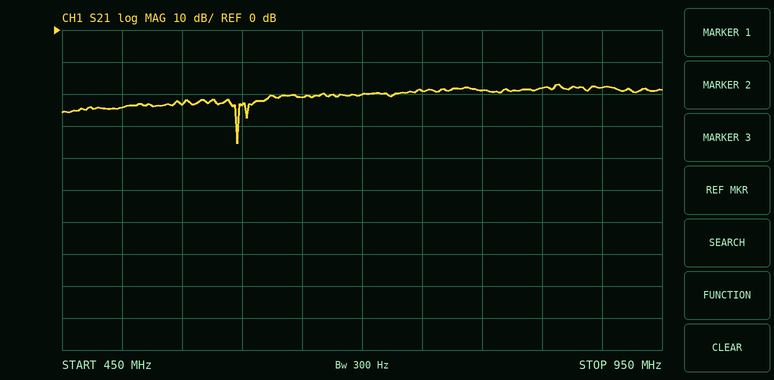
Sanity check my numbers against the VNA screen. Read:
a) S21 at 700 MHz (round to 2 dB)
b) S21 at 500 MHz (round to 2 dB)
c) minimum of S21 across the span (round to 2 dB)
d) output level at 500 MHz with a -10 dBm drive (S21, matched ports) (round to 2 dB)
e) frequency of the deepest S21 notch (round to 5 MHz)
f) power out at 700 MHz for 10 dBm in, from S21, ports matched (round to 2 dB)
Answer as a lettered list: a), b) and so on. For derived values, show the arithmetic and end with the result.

a) -20 dB
b) -24 dB
c) -36 dB
d) -10 dBm + (-24 dB) = -34 dBm
e) 595 MHz
f) 10 dBm + (-20 dB) = -10 dBm
